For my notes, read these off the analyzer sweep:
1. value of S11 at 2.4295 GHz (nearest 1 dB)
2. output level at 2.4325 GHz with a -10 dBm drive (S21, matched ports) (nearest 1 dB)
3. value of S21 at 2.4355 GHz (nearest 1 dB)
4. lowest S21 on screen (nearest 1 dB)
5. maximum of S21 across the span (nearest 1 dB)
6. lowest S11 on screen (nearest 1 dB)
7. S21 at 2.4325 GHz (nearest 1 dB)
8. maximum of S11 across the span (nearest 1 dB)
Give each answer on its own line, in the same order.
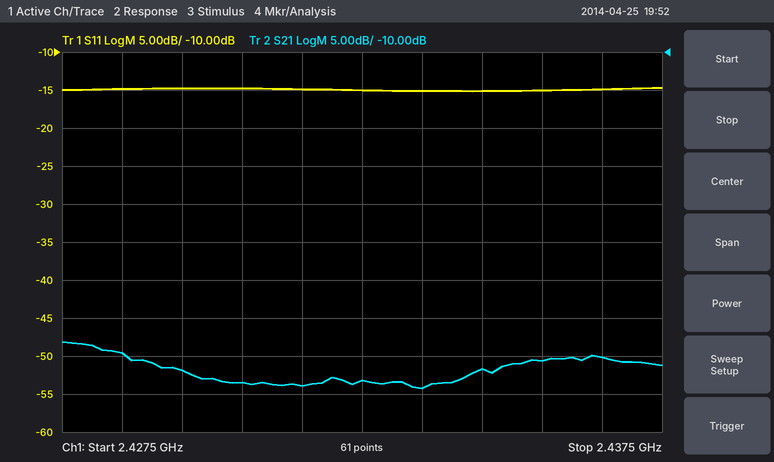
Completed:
-15 dB
-63 dBm
-51 dB
-54 dB
-48 dB
-15 dB
-53 dB
-15 dB
